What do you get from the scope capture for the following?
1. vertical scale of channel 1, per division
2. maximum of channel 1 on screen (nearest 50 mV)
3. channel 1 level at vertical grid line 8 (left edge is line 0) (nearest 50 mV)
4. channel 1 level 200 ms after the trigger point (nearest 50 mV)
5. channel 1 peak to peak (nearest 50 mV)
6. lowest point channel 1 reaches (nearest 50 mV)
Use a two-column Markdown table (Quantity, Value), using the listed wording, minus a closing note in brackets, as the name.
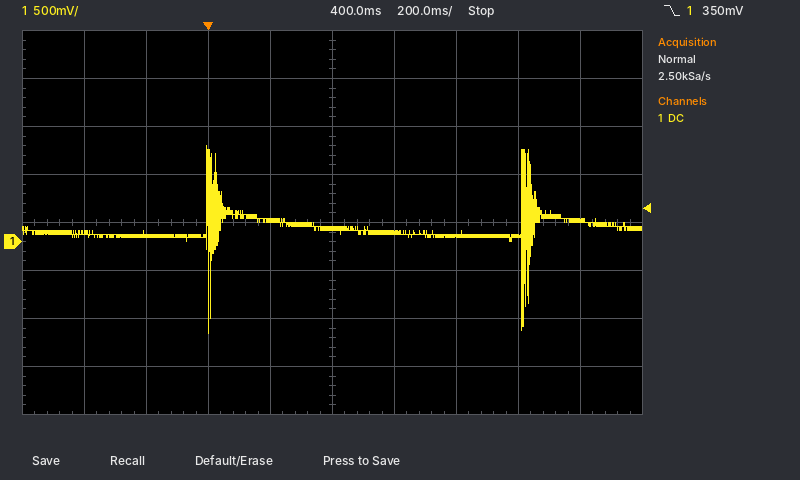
| Quantity | Value |
|---|---|
| vertical scale of channel 1, per division | 500 mV |
| maximum of channel 1 on screen | 1.00 V |
| channel 1 level at vertical grid line 8 (left edge is line 0) | 50 mV |
| channel 1 level 200 ms after the trigger point | 200 mV |
| channel 1 peak to peak | 1.95 V |
| lowest point channel 1 reaches | -950 mV |
